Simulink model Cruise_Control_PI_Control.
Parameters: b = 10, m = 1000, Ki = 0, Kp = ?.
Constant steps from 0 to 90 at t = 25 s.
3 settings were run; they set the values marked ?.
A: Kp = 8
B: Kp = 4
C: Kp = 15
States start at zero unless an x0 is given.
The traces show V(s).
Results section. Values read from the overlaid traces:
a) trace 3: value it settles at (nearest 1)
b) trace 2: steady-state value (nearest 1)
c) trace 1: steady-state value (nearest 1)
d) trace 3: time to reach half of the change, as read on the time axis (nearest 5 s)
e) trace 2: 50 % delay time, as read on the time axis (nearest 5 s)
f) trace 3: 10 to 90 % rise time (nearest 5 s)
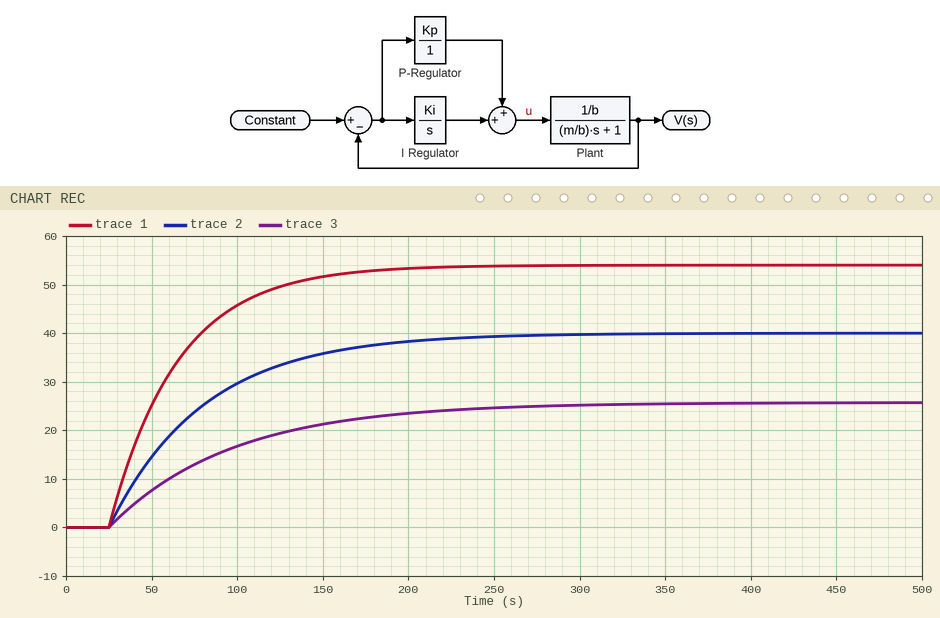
26
40
54
75 s
65 s
155 s
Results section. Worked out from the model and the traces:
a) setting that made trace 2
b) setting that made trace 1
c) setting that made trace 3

A
C
B
